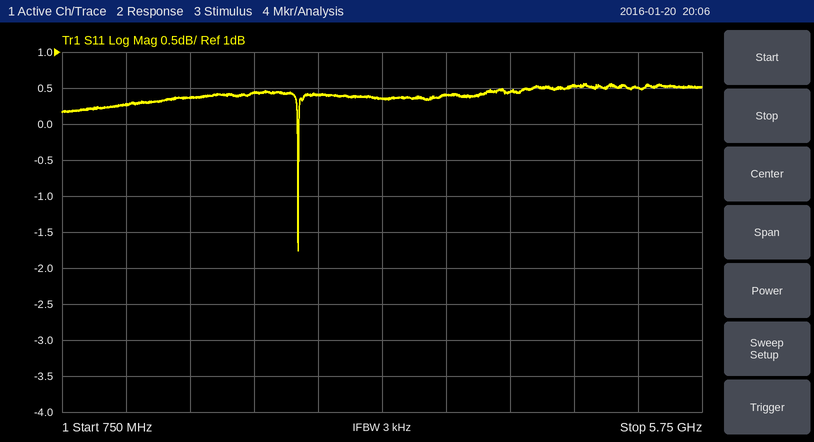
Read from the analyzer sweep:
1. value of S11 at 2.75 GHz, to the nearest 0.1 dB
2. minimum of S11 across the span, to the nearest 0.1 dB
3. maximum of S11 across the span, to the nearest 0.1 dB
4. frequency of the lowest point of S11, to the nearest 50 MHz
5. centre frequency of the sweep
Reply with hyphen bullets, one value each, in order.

- 0.4 dB
- -1.8 dB
- 0.6 dB
- 2.60 GHz
- 3.25 GHz
